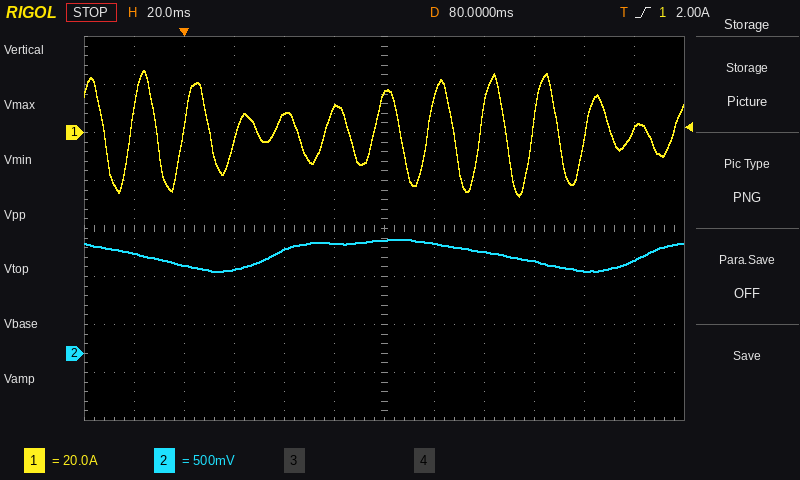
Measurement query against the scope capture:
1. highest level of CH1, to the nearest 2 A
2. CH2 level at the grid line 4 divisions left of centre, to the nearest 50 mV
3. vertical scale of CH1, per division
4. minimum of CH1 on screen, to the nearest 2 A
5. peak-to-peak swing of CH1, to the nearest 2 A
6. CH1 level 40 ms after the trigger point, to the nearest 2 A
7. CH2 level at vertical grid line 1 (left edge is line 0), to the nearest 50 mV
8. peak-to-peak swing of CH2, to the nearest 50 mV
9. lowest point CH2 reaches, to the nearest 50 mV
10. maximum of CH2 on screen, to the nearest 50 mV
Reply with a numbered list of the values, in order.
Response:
1. 26 A
2. 900 mV
3. 20 A
4. -26 A
5. 52 A
6. 8 A
7. 1.05 V
8. 350 mV
9. 850 mV
10. 1.20 V
